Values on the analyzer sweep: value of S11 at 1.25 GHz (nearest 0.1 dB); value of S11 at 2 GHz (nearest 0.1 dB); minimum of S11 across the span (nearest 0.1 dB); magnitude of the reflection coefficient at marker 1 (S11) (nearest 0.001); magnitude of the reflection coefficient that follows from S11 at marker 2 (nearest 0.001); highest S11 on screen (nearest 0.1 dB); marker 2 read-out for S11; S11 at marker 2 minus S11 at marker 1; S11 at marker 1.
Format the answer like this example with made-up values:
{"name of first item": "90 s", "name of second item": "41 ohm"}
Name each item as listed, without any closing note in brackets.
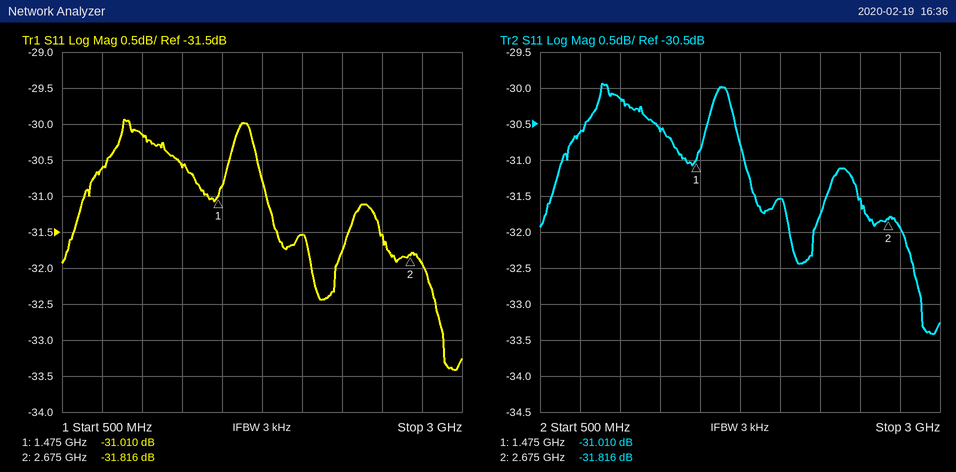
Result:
{"value of S11 at 1.25 GHz": "-30.6 dB", "value of S11 at 2 GHz": "-31.5 dB", "minimum of S11 across the span": "-33.4 dB", "magnitude of the reflection coefficient at marker 1 (S11)": "0.028", "magnitude of the reflection coefficient that follows from S11 at marker 2": "0.026", "highest S11 on screen": "-29.9 dB", "marker 2 read-out for S11": "-31.816 dB", "S11 at marker 2 minus S11 at marker 1": "-0.806 dB", "S11 at marker 1": "-31.010 dB"}
